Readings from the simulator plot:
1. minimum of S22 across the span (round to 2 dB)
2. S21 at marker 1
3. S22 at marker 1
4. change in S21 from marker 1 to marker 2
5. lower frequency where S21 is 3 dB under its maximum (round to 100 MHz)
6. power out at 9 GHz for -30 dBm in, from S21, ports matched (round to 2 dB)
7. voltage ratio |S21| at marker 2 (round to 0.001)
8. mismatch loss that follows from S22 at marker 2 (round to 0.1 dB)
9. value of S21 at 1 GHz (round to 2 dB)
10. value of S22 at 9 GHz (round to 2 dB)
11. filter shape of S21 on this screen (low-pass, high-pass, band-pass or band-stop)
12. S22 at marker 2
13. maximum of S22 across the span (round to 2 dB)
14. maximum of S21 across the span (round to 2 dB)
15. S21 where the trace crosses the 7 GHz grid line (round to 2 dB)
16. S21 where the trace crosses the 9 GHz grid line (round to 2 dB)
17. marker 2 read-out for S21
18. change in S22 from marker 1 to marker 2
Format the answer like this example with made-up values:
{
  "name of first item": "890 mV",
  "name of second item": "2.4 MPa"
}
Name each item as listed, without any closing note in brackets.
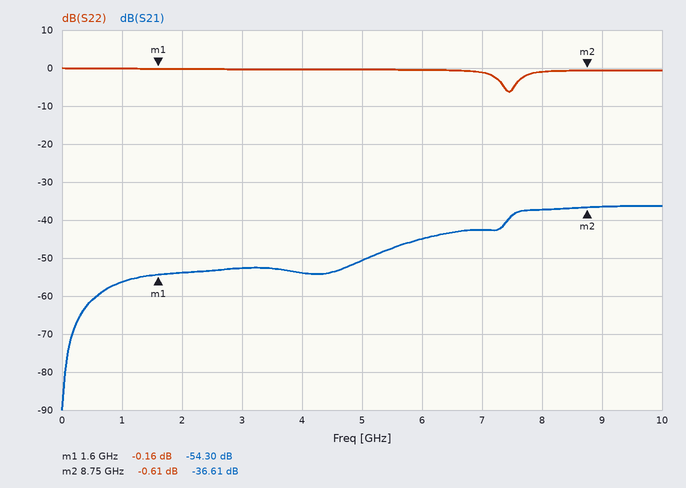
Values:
{
  "minimum of S22 across the span": "-6 dB",
  "S21 at marker 1": "-54.30 dB",
  "S22 at marker 1": "-0.16 dB",
  "change in S21 from marker 1 to marker 2": "17.69 dB",
  "lower frequency where S21 is 3 dB under its maximum": "7.5 GHz",
  "power out at 9 GHz for -30 dBm in, from S21, ports matched": "-66 dBm",
  "voltage ratio |S21| at marker 2": "0.015",
  "mismatch loss that follows from S22 at marker 2": "8.8 dB",
  "value of S21 at 1 GHz": "-56 dB",
  "value of S22 at 9 GHz": "0 dB",
  "filter shape of S21 on this screen": "high-pass",
  "S22 at marker 2": "-0.61 dB",
  "maximum of S22 across the span": "0 dB",
  "maximum of S21 across the span": "-36 dB",
  "S21 where the trace crosses the 7 GHz grid line": "-42 dB",
  "S21 where the trace crosses the 9 GHz grid line": "-36 dB",
  "marker 2 read-out for S21": "-36.61 dB",
  "change in S22 from marker 1 to marker 2": "-0.45 dB"
}
